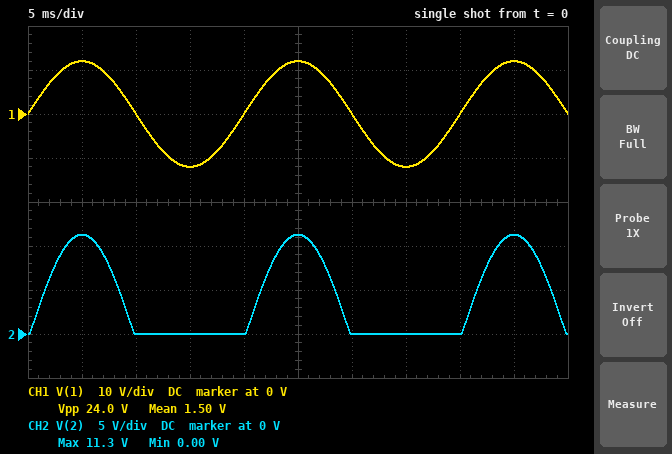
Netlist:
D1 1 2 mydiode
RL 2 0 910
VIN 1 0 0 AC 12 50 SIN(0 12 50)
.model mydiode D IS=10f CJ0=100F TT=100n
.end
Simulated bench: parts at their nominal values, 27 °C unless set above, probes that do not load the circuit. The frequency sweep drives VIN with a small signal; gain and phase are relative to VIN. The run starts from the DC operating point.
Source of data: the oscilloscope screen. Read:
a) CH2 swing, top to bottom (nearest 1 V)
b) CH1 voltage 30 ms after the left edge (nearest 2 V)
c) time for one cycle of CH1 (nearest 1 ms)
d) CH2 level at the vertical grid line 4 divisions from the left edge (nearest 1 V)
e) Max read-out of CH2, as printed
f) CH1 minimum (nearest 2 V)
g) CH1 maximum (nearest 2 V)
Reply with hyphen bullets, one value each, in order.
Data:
- 11 V
- 0 V
- 20 ms
- 0 V
- 11.3 V
- -12 V
- 12 V
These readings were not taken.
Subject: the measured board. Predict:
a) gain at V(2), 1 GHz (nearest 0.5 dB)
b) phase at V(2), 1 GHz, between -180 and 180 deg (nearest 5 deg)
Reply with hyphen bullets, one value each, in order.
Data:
- -6.0 dB
- 60 deg
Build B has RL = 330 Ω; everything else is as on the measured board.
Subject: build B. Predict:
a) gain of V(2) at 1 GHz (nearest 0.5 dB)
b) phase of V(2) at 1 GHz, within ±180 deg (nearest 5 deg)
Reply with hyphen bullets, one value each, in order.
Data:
- -14.0 dB
- 80 deg
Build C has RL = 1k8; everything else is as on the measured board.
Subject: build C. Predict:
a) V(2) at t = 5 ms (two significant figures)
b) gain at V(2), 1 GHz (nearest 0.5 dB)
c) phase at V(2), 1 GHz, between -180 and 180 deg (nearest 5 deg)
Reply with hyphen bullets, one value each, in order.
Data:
- 11 V
- -2.5 dB
- 40 deg
